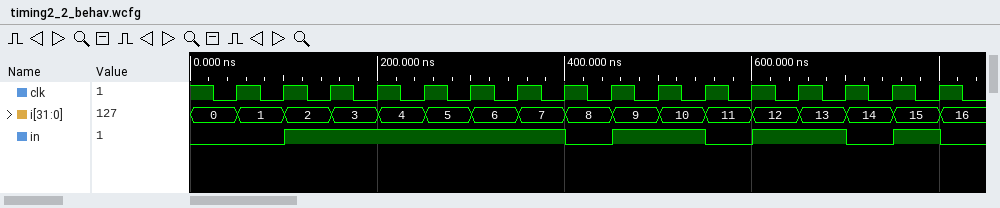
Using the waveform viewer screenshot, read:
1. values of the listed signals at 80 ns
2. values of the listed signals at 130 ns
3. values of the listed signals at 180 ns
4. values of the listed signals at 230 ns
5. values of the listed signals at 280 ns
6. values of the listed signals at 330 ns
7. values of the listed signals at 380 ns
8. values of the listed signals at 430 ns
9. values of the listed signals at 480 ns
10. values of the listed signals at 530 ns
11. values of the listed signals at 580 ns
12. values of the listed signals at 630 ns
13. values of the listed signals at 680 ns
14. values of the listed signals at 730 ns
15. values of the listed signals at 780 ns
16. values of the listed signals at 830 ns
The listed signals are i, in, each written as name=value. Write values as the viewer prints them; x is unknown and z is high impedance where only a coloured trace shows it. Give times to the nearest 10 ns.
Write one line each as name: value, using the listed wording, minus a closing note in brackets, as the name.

values of the listed signals at 80 ns: i=1, in=0
values of the listed signals at 130 ns: i=2, in=1
values of the listed signals at 180 ns: i=3, in=1
values of the listed signals at 230 ns: i=4, in=1
values of the listed signals at 280 ns: i=5, in=1
values of the listed signals at 330 ns: i=6, in=1
values of the listed signals at 380 ns: i=7, in=1
values of the listed signals at 430 ns: i=8, in=0
values of the listed signals at 480 ns: i=9, in=1
values of the listed signals at 530 ns: i=10, in=1
values of the listed signals at 580 ns: i=11, in=0
values of the listed signals at 630 ns: i=12, in=1
values of the listed signals at 680 ns: i=13, in=1
values of the listed signals at 730 ns: i=14, in=0
values of the listed signals at 780 ns: i=15, in=1
values of the listed signals at 830 ns: i=16, in=0
